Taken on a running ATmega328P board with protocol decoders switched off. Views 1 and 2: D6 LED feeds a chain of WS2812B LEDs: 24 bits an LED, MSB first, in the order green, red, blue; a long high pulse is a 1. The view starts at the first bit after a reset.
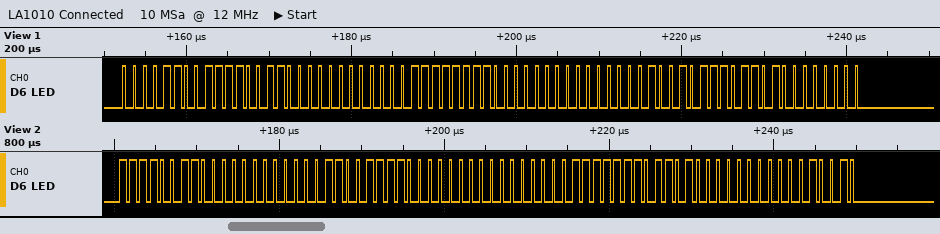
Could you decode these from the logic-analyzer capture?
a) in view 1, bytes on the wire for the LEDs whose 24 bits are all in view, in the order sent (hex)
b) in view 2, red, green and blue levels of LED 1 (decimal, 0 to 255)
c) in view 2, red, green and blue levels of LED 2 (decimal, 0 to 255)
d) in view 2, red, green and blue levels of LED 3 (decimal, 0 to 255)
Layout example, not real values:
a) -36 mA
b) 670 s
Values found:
a) 0C F3 00 0F F0 00 12 ED 00
b) 0, 243, 12
c) 0, 240, 15
d) 0, 237, 18
